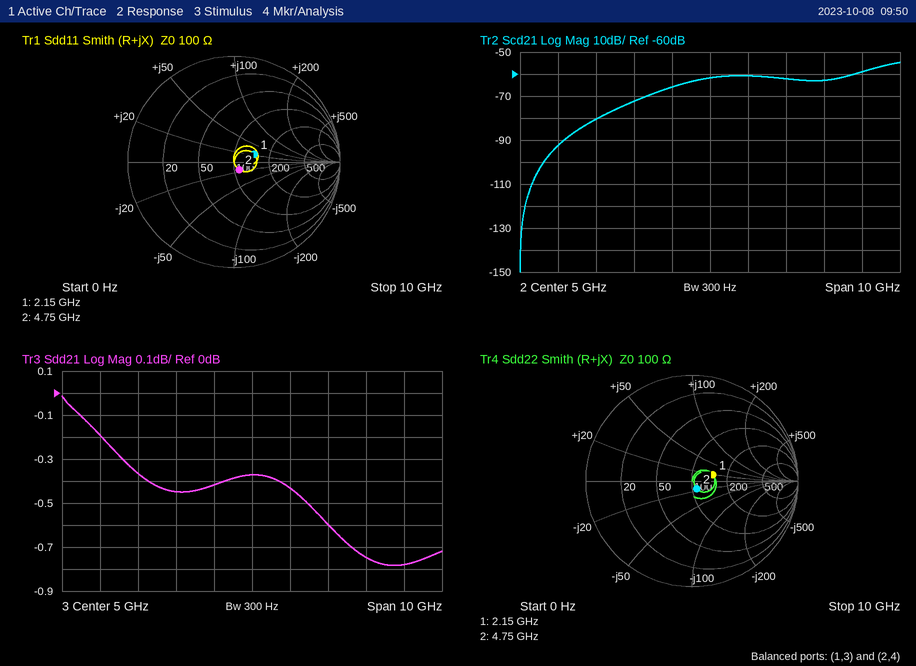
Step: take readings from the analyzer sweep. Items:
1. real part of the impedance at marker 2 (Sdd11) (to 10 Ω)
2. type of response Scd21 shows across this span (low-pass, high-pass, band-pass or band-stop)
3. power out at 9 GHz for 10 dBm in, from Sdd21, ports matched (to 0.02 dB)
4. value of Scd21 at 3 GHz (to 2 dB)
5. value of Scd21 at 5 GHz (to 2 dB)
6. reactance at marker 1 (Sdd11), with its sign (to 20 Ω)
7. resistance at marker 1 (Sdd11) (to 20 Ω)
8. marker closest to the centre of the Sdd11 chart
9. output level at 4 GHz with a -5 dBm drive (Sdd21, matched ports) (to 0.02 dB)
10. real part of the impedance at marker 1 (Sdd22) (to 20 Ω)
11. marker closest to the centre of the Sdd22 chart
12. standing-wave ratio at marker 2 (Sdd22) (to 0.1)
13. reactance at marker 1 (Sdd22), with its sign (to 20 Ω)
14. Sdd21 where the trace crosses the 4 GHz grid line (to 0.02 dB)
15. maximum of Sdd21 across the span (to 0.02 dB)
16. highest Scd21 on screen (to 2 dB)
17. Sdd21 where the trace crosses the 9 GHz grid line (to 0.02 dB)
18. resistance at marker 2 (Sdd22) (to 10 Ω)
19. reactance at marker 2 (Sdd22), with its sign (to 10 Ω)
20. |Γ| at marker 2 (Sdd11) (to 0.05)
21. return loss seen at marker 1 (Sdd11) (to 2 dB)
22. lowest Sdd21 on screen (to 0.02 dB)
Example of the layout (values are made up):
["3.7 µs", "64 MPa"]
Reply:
["110 Ω", "high-pass", "9.22 dBm", "-72 dB", "-62 dB", "+20 Ω", "140 Ω", "marker 2", "-5.42 dBm", "140 Ω", "marker 2", "1.2", "+20 Ω", "-0.42 dB", "-0.02 dB", "-54 dB", "-0.78 dB", "110 Ω", "-20 Ω", "0.10", "14 dB", "-0.78 dB"]
